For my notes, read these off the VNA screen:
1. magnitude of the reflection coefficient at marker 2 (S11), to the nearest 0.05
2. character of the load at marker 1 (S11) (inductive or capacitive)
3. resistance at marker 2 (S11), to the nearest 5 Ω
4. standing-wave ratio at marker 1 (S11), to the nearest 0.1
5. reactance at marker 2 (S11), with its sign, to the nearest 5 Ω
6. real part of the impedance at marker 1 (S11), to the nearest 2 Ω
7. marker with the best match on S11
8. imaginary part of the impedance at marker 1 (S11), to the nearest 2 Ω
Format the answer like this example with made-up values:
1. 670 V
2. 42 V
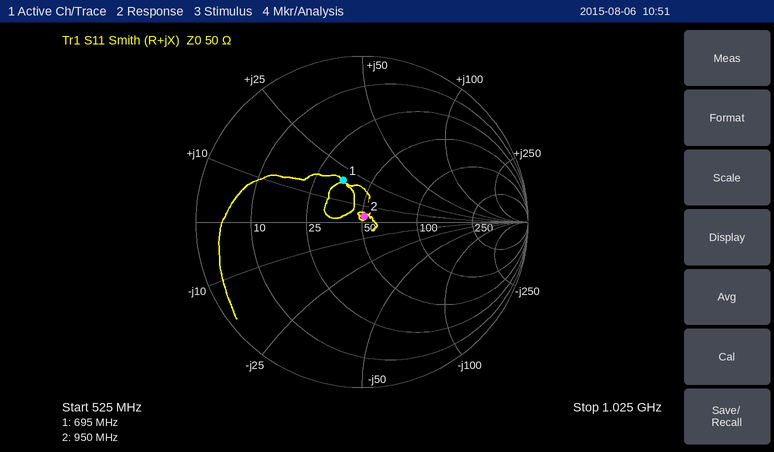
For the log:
1. 0.05
2. inductive
3. 50 Ω
4. 1.8
5. +5 Ω
6. 36 Ω
7. marker 2
8. +20 Ω
